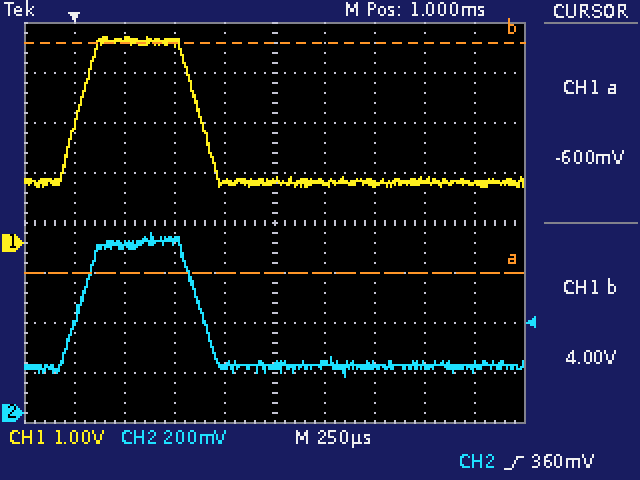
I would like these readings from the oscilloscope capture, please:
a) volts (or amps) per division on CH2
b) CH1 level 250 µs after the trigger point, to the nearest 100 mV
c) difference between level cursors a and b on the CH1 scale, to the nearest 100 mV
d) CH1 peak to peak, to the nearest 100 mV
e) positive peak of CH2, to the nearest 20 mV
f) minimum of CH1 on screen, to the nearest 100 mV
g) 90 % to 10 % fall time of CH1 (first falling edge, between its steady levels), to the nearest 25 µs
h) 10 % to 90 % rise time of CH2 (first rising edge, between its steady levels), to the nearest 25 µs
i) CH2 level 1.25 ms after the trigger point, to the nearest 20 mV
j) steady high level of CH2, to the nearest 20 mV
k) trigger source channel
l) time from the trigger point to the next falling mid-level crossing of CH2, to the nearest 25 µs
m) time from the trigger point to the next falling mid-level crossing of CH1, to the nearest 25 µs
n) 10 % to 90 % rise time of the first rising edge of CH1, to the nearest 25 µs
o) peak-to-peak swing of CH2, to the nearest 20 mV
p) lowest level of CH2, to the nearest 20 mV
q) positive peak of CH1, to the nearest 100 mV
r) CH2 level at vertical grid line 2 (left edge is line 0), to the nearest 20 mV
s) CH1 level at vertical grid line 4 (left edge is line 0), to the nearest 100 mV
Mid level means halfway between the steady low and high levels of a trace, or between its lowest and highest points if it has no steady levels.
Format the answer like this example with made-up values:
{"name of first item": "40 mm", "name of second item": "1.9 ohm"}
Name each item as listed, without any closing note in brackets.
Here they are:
{"volts (or amps) per division on CH2": "200 mV", "CH1 level 250 µs after the trigger point, to the nearest 100 mV": "4.1 V", "difference between level cursors a and b on the CH1 scale, to the nearest 100 mV": "4.6 V", "CH1 peak to peak, to the nearest 100 mV": "3.0 V", "positive peak of CH2, to the nearest 20 mV": "720 mV", "minimum of CH1 on screen, to the nearest 100 mV": "1.1 V", "90 % to 10 % fall time of CH1 (first falling edge, between its steady levels), to the nearest 25 µs": "175 µs", "10 % to 90 % rise time of CH2 (first rising edge, between its steady levels), to the nearest 25 µs": "150 µs", "CH2 level 1.25 ms after the trigger point, to the nearest 20 mV": "200 mV", "steady high level of CH2, to the nearest 20 mV": "680 mV", "trigger source channel": "CH2", "time from the trigger point to the next falling mid-level crossing of CH2, to the nearest 25 µs": "625 µs", "time from the trigger point to the next falling mid-level crossing of CH1, to the nearest 25 µs": "625 µs", "10 % to 90 % rise time of the first rising edge of CH1, to the nearest 25 µs": "150 µs", "peak-to-peak swing of CH2, to the nearest 20 mV": "580 mV", "lowest level of CH2, to the nearest 20 mV": "140 mV", "positive peak of CH1, to the nearest 100 mV": "4.1 V", "CH2 level at vertical grid line 2 (left edge is line 0), to the nearest 20 mV": "680 mV", "CH1 level at vertical grid line 4 (left edge is line 0), to the nearest 100 mV": "1.2 V"}
